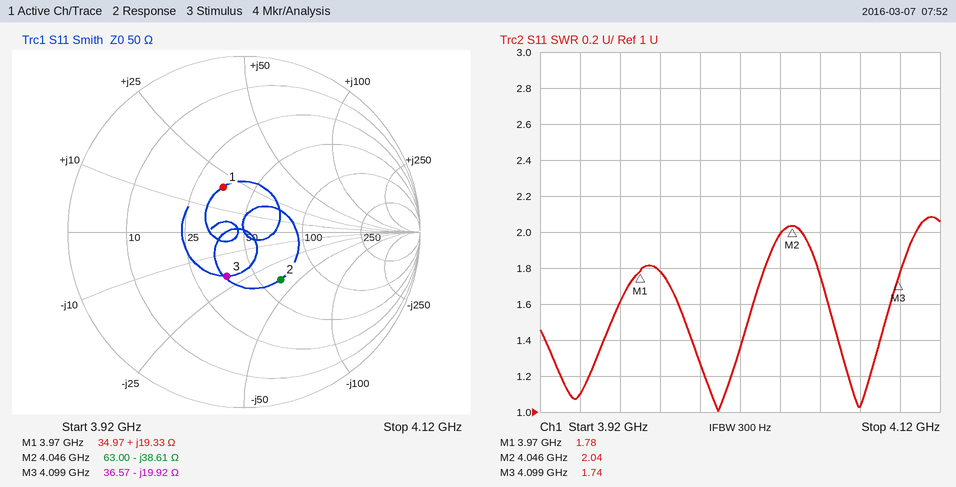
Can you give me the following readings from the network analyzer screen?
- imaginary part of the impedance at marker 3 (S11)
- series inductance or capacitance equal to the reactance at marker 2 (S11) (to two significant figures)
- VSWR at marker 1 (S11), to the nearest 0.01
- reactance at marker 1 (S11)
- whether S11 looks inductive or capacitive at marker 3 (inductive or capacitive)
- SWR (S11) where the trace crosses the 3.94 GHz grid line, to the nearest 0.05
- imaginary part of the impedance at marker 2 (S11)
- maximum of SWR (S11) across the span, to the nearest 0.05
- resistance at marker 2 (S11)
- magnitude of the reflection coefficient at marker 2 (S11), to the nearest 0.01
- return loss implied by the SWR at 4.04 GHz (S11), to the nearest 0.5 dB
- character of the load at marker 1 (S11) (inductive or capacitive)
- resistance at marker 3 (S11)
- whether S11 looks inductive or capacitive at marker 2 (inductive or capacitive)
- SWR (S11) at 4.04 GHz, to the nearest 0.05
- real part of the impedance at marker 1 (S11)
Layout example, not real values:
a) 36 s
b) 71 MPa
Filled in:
a) -19.92 Ω
b) 1.0 pF
c) 1.78
d) +19.33 Ω
e) capacitive
f) 1.10
g) -38.61 Ω
h) 2.10
i) 63.00 Ω
j) 0.34
k) 9.5 dB
l) inductive
m) 36.57 Ω
n) capacitive
o) 2.00
p) 34.97 Ω
